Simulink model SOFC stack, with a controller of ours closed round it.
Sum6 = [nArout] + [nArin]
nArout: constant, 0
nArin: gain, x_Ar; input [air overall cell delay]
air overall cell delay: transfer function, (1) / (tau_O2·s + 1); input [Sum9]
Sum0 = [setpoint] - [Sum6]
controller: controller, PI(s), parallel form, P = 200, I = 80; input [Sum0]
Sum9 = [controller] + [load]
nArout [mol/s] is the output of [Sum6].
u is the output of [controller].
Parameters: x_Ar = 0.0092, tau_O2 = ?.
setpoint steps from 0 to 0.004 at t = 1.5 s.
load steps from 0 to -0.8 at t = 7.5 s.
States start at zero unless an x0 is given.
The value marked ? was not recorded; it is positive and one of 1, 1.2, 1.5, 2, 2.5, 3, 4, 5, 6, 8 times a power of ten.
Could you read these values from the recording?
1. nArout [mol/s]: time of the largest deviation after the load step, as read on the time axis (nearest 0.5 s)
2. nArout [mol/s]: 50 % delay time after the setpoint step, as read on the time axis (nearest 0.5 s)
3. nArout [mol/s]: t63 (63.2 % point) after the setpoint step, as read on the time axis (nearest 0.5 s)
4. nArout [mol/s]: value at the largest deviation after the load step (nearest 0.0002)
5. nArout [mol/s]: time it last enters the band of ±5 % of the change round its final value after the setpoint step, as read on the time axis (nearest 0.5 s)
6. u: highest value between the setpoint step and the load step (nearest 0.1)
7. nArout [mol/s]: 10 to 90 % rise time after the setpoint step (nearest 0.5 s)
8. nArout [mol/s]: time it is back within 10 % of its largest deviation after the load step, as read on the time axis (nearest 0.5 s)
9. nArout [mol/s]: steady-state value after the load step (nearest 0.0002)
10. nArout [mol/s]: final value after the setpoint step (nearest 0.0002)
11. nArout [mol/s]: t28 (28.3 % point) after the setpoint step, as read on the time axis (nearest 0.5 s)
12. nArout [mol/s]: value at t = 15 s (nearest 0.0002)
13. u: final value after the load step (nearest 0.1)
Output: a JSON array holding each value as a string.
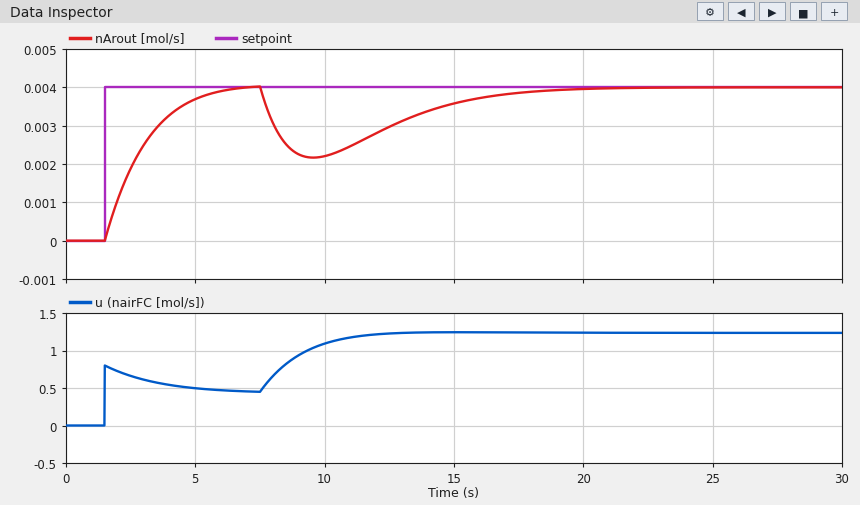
["9.5 s", "2.5 s", "3.0 s", "0.0022", "5.5 s", "0.8", "3.0 s", "17.0 s", "0.0040", "0.0040", "2.0 s", "0.0036", "1.2"]
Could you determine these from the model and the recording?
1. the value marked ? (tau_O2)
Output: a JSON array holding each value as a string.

["3"]
